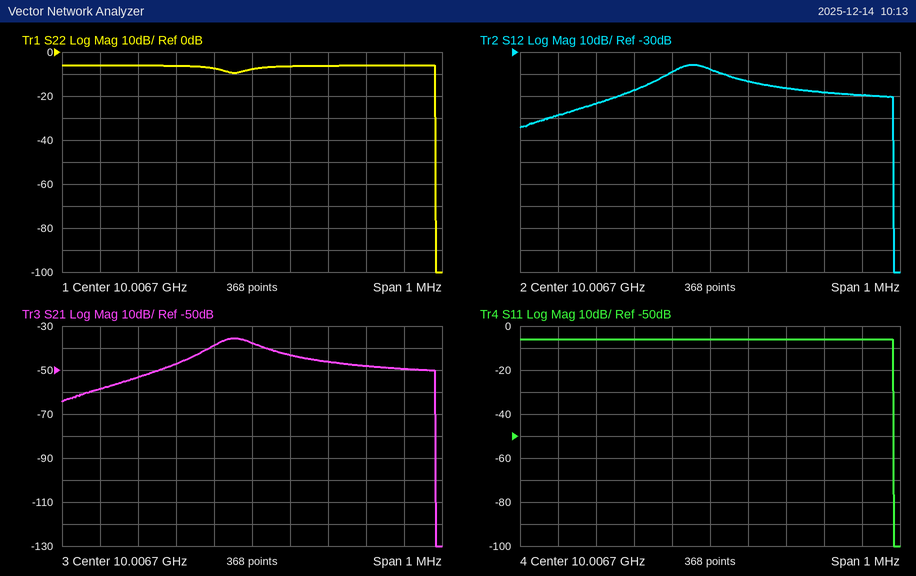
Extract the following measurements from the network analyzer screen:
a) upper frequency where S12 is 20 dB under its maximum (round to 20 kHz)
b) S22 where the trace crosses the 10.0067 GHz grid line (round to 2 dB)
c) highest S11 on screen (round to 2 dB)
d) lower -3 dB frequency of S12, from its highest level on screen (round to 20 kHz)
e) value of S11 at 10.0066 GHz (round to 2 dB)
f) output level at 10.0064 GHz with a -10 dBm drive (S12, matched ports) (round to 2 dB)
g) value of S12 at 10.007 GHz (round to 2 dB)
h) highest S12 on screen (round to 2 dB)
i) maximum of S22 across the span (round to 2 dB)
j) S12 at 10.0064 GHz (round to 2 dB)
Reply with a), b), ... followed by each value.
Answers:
a) 10.00718 GHz
b) -8 dB
c) -6 dB
d) 10.00660 GHz
e) -6 dB
f) -64 dBm
g) -48 dB
h) -36 dB
i) -6 dB
j) -54 dB
